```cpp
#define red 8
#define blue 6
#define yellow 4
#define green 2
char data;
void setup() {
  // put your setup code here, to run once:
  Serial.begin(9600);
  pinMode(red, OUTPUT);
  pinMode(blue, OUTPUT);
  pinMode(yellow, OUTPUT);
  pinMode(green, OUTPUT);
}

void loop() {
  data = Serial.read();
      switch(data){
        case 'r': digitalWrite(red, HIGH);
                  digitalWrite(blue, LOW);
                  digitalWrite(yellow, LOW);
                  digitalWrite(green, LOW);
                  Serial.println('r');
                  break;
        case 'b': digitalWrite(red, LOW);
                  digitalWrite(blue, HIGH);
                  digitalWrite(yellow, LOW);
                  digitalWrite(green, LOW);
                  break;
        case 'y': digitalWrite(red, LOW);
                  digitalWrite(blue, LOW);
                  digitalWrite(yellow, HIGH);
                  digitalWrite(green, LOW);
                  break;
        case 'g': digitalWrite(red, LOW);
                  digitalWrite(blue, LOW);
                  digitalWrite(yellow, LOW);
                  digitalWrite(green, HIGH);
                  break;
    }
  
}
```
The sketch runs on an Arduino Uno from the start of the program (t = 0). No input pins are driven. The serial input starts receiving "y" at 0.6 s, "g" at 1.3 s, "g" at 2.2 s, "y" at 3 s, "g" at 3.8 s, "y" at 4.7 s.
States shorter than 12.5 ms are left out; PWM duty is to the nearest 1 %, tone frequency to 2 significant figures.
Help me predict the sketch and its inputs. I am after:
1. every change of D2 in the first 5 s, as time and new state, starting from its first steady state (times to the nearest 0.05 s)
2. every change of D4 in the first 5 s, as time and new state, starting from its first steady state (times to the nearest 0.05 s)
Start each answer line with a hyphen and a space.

- 0 s low; 1.3 s high; 3 s low; 3.8 s high; 4.7 s low
- 0 s low; 0.6 s high; 1.3 s low; 3 s high; 3.8 s low; 4.7 s high
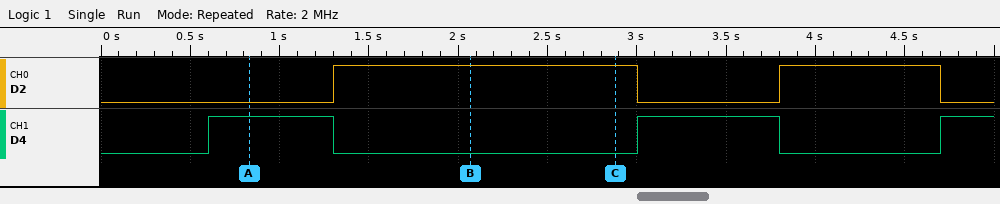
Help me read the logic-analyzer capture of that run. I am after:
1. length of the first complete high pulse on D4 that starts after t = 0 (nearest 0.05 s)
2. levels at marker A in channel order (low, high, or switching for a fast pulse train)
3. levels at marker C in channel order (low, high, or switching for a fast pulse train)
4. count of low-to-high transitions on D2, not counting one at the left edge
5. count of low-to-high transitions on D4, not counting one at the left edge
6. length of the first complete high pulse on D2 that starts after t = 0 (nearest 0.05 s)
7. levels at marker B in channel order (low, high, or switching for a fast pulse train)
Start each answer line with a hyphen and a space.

- 0.70 s
- D2 low, D4 high
- D2 high, D4 low
- 2
- 3
- 1.70 s
- D2 high, D4 low
